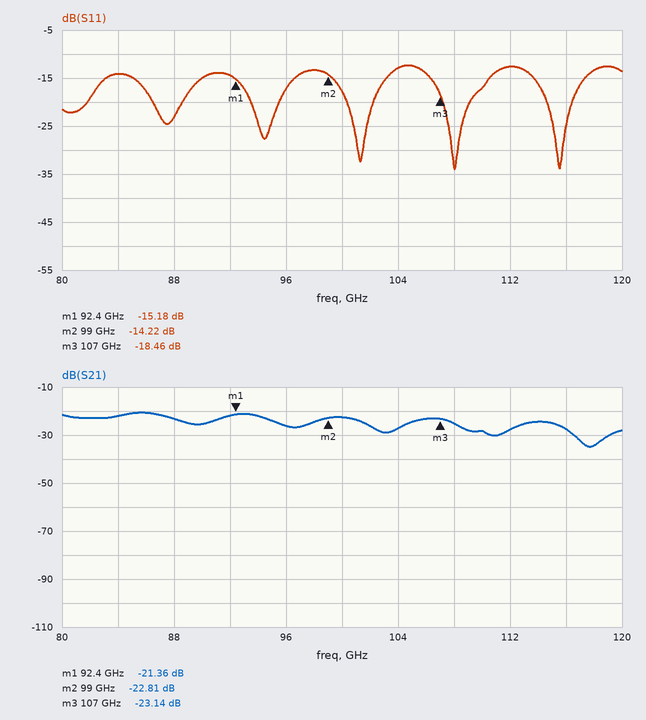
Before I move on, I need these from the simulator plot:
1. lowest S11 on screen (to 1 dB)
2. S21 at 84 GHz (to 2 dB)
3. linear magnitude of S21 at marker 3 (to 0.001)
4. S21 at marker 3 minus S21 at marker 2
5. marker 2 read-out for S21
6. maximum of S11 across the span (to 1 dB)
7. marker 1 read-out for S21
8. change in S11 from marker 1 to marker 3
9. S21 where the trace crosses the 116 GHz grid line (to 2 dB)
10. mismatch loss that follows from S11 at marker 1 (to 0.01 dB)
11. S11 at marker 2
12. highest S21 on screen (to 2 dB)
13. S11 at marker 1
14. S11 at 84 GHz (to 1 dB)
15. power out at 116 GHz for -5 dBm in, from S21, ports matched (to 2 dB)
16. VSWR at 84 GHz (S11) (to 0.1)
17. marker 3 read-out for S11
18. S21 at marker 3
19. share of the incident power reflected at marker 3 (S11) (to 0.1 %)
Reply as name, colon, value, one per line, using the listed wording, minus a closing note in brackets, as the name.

lowest S11 on screen: -34 dB
S21 at 84 GHz: -22 dB
linear magnitude of S21 at marker 3: 0.070
S21 at marker 3 minus S21 at marker 2: -0.33 dB
marker 2 read-out for S21: -22.81 dB
maximum of S11 across the span: -12 dB
marker 1 read-out for S21: -21.36 dB
change in S11 from marker 1 to marker 3: -3.28 dB
S21 where the trace crosses the 116 GHz grid line: -28 dB
mismatch loss that follows from S11 at marker 1: 0.13 dB
S11 at marker 2: -14.22 dB
highest S21 on screen: -20 dB
S11 at marker 1: -15.18 dB
S11 at 84 GHz: -14 dB
power out at 116 GHz for -5 dBm in, from S21, ports matched: -32 dBm
VSWR at 84 GHz (S11): 1.5
marker 3 read-out for S11: -18.46 dB
S21 at marker 3: -23.14 dB
share of the incident power reflected at marker 3 (S11): 1.4 %
